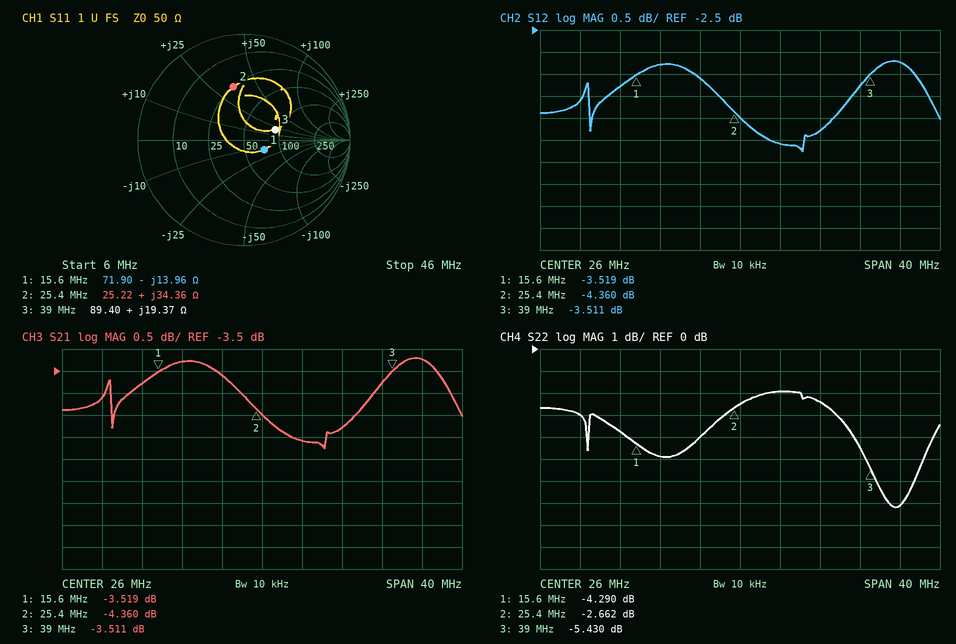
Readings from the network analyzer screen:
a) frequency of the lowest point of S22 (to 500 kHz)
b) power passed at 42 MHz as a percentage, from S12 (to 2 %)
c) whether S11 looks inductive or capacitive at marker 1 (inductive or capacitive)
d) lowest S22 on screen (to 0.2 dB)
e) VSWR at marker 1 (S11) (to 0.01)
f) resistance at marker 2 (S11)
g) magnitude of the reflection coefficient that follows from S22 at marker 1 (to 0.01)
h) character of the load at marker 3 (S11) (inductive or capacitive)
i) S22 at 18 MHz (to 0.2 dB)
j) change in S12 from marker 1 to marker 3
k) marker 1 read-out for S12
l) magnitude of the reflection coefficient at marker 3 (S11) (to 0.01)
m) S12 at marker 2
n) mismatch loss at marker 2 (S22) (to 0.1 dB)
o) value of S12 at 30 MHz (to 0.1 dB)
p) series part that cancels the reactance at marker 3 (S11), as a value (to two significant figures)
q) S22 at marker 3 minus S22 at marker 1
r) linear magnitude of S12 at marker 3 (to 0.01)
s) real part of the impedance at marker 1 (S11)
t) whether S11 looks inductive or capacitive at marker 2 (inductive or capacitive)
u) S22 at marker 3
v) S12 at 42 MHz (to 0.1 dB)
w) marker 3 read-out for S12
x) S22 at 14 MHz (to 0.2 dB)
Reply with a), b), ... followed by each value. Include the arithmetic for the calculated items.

a) 41.5 MHz
b) 10^(-3.2/10) ≈ 48 %
c) capacitive
d) -7.2 dB
e) 1.54
f) 25.22 Ω
g) 10^(-4.29/20) ≈ 0.61
h) inductive
i) -4.8 dB
j) -3.511 − (-3.519) = 0.008 dB
k) -3.519 dB
l) 0.31
m) -4.360 dB
n) −10 log10(1 − 10^(-2.662/10)) ≈ 3.4 dB
o) -5.1 dB
p) C = 1/(2π × 39 MHz × 19.37 Ω) ≈ 211 pF, so 210 pF to two significant figures
q) -5.43 − (-4.29) = -1.140 dB
r) 10^(-3.511/20) ≈ 0.67
s) 71.90 Ω
t) inductive
u) -5.430 dB
v) -3.2 dB
w) -3.511 dB
x) -3.8 dB
